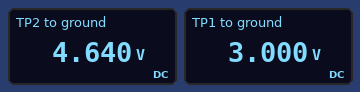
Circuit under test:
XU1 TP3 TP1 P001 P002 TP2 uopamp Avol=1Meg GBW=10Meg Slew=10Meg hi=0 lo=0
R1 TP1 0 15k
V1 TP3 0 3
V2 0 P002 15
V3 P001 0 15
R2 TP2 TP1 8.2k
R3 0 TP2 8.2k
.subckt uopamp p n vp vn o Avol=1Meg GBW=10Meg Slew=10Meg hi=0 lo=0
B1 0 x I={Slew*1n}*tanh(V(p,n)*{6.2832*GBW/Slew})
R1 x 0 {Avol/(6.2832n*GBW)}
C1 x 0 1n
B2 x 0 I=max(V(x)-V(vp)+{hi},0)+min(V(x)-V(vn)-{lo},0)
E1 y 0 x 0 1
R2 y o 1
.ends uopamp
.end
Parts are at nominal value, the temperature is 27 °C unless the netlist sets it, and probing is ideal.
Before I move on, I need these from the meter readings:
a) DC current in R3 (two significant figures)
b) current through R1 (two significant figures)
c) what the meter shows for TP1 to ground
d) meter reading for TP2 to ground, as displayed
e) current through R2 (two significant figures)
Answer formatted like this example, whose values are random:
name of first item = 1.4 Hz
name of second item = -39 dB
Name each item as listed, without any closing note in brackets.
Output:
DC current in R3 = 570 µA
current through R1 = 200 µA
what the meter shows for TP1 to ground = 3.000 V
meter reading for TP2 to ground, as displayed = 4.640 V
current through R2 = 200 µA
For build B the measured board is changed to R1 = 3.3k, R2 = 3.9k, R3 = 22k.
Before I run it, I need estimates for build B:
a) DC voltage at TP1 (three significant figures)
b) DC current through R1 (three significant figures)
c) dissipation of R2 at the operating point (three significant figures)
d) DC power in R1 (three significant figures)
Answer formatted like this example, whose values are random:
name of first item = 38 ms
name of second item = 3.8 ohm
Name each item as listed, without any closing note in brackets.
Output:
DC voltage at TP1 = 3.00 V
DC current through R1 = 909 µA
dissipation of R2 at the operating point = 3.22 mW
DC power in R1 = 2.73 mW
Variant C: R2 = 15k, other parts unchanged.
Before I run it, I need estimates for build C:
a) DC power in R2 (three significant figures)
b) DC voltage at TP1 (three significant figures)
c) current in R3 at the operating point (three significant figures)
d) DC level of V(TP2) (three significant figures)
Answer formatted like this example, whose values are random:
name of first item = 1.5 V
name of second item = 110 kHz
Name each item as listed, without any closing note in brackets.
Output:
DC power in R2 = 600 µW
DC voltage at TP1 = 3.00 V
current in R3 at the operating point = 732 µA
DC level of V(TP2) = 6.00 V
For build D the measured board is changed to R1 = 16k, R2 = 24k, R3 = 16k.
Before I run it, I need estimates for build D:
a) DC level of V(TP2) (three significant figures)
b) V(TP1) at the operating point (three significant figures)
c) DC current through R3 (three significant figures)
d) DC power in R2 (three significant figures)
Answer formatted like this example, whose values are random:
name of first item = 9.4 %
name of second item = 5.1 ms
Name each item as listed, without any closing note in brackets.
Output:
DC level of V(TP2) = 7.50 V
V(TP1) at the operating point = 3.00 V
DC current through R3 = 469 µA
DC power in R2 = 844 µW
